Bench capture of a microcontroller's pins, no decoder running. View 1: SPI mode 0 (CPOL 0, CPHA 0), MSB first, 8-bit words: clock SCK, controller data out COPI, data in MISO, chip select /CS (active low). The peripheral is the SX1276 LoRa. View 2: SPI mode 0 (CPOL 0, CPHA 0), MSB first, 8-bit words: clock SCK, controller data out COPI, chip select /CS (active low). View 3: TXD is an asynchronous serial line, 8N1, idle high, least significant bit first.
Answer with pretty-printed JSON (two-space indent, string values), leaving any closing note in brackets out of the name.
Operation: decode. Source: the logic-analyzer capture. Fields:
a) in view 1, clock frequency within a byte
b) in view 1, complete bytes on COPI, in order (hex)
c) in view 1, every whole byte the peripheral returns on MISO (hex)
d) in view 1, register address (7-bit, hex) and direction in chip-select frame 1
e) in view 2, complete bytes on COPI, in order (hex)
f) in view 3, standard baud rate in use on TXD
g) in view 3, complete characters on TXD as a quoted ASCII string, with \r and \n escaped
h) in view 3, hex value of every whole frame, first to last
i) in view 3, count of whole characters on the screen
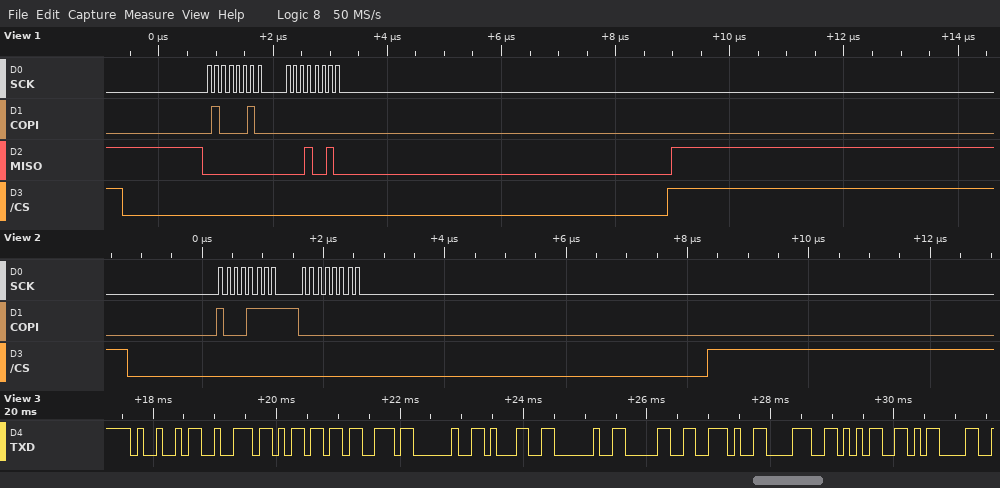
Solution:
{
  "in view 1, clock frequency within a byte": "8 MHz",
  "in view 1, complete bytes on COPI, in order": "42 00",
  "in view 1, every whole byte the peripheral returns on MISO": "00 12",
  "in view 1, register address (7-bit, hex) and direction in chip-select frame 1": "0x42 read",
  "in view 2, complete bytes on COPI, in order": "8F 00",
  "in view 3, standard baud rate in use on TXD": "9600 baud",
  "in view 3, complete characters on TXD as a quoted ASCII string, with \\r and \\n escaped": "\"Irms 1 0.85\\r\"",
  "in view 3, hex value of every whole frame, first to last": "0x49 0x72 0x6D 0x73 0x20 0x31 0x20 0x30 0x2E 0x38 0x35 0x0D",
  "in view 3, count of whole characters on the screen": "12"
}
